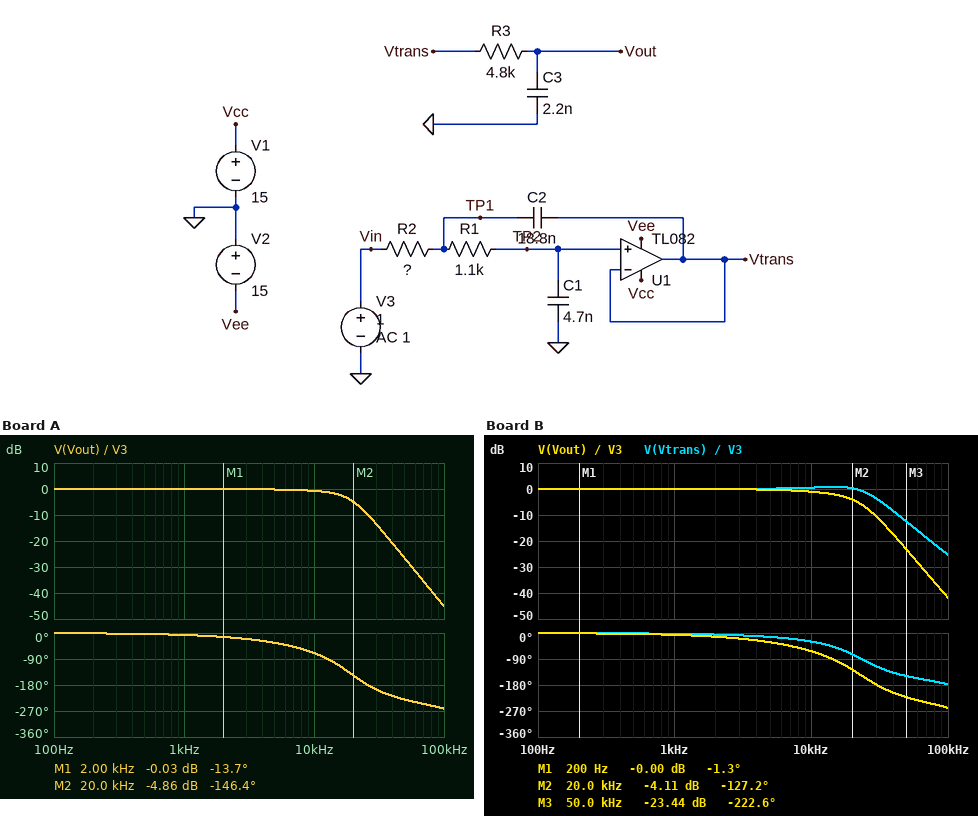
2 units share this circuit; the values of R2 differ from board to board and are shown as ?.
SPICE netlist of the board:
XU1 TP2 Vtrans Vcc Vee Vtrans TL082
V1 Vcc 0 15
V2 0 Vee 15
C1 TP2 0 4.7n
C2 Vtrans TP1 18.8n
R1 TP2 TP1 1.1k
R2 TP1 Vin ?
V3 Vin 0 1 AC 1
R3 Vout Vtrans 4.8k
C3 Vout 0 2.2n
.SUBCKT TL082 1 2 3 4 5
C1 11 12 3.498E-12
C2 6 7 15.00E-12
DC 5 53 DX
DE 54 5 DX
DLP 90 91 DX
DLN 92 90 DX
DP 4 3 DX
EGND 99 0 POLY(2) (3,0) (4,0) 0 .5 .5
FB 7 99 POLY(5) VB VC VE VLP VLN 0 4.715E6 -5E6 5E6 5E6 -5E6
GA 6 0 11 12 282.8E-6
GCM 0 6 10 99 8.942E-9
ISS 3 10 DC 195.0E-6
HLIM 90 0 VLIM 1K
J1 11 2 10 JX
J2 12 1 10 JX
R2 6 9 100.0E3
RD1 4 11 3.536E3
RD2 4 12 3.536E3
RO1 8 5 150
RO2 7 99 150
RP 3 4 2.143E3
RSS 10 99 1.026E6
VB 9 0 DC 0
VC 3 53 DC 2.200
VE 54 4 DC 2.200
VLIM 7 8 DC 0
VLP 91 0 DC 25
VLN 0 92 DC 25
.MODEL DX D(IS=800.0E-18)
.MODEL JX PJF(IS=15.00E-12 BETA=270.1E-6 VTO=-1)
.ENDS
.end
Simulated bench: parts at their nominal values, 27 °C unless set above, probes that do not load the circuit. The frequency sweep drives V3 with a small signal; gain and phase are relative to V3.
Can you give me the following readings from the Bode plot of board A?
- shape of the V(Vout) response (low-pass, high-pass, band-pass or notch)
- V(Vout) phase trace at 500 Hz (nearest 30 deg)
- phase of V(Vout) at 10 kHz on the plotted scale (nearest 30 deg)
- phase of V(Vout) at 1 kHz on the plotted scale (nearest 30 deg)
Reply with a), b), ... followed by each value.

a) low-pass
b) 0 deg
c) -60 deg
d) 0 deg
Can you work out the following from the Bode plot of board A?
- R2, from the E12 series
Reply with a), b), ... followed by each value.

a) 680 Ω
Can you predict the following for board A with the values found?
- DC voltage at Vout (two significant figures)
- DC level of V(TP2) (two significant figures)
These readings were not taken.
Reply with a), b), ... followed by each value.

a) 1.0 V
b) 1.0 V
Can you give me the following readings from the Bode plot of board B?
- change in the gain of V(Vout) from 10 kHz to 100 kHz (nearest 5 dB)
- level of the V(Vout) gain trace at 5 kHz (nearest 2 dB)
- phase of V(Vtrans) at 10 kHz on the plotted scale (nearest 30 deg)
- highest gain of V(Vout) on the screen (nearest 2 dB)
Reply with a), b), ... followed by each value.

a) -40 dB
b) 0 dB
c) -30 deg
d) 0 dB
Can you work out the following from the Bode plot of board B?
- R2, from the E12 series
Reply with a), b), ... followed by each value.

a) 470 Ω
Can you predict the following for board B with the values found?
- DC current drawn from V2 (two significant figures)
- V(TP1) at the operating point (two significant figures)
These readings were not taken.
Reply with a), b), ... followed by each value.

a) 14 mA
b) 1.0 V
